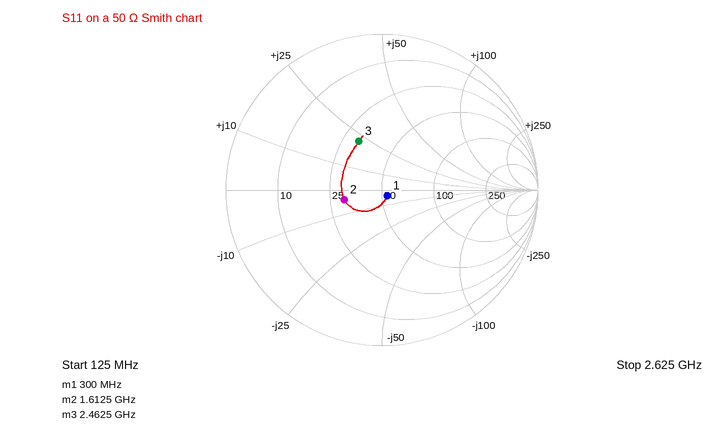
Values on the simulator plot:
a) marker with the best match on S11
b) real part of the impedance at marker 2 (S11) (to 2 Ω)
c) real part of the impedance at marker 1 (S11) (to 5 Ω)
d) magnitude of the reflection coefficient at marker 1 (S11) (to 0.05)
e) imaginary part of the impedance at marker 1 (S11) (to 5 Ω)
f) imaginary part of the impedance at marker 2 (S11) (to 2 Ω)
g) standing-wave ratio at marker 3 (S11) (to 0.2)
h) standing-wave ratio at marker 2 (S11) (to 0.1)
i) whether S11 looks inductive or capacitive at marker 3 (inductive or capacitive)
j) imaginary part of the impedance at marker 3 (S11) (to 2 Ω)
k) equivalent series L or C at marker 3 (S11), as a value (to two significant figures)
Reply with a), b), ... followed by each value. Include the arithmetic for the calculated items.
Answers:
a) marker 1
b) 30 Ω
c) 55 Ω
d) 0.05
e) -5 Ω
f) -4 Ω
g) 2.0
h) 1.7
i) inductive
j) +22 Ω
k) L = 22 Ω/(2π × 2.4625 GHz) ≈ 1.4 nH
